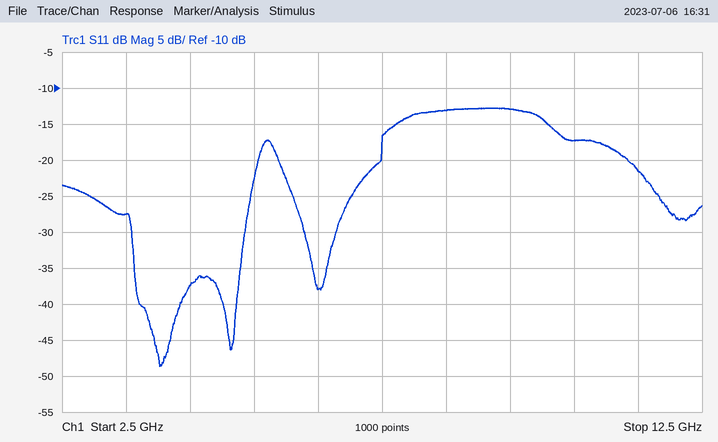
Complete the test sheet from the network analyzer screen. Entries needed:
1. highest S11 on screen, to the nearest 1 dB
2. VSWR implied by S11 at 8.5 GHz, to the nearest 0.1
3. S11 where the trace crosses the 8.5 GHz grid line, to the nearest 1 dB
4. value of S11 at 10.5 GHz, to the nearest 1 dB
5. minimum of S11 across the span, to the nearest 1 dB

-13 dB
1.6
-13 dB
-17 dB
-49 dB
